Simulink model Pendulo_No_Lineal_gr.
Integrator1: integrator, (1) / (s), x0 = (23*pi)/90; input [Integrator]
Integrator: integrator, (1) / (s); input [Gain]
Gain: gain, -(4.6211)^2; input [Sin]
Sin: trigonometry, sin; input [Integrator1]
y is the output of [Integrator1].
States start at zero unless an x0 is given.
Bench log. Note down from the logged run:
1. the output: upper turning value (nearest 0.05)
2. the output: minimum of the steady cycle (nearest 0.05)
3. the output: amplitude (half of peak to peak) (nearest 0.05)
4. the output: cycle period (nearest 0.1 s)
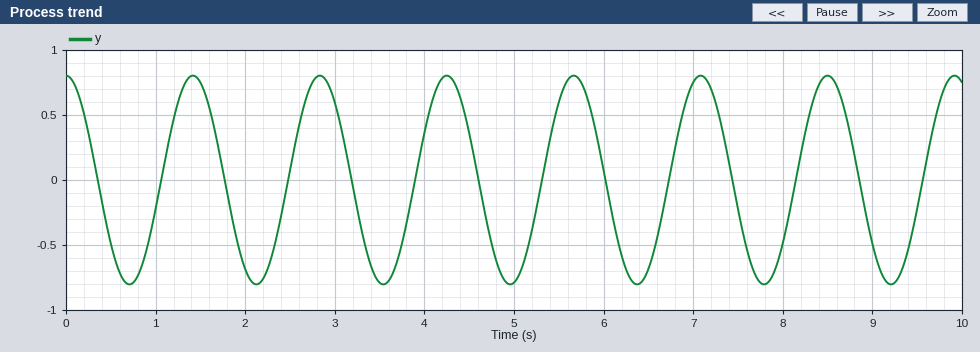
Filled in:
0.80
-0.80
0.80
1.4 s
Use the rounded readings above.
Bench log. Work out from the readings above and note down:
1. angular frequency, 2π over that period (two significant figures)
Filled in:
4.5 rad/s
